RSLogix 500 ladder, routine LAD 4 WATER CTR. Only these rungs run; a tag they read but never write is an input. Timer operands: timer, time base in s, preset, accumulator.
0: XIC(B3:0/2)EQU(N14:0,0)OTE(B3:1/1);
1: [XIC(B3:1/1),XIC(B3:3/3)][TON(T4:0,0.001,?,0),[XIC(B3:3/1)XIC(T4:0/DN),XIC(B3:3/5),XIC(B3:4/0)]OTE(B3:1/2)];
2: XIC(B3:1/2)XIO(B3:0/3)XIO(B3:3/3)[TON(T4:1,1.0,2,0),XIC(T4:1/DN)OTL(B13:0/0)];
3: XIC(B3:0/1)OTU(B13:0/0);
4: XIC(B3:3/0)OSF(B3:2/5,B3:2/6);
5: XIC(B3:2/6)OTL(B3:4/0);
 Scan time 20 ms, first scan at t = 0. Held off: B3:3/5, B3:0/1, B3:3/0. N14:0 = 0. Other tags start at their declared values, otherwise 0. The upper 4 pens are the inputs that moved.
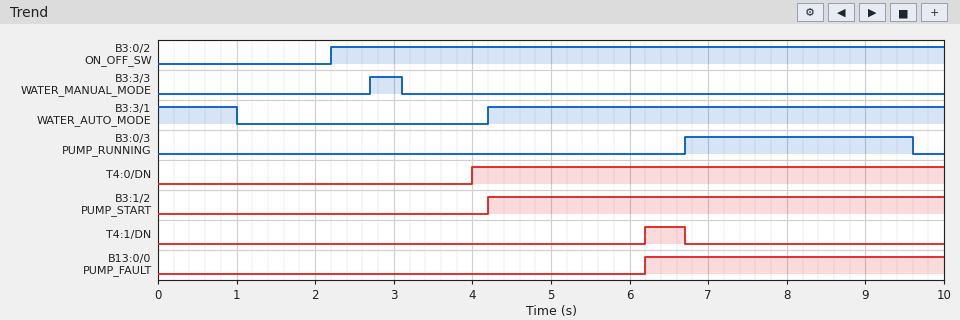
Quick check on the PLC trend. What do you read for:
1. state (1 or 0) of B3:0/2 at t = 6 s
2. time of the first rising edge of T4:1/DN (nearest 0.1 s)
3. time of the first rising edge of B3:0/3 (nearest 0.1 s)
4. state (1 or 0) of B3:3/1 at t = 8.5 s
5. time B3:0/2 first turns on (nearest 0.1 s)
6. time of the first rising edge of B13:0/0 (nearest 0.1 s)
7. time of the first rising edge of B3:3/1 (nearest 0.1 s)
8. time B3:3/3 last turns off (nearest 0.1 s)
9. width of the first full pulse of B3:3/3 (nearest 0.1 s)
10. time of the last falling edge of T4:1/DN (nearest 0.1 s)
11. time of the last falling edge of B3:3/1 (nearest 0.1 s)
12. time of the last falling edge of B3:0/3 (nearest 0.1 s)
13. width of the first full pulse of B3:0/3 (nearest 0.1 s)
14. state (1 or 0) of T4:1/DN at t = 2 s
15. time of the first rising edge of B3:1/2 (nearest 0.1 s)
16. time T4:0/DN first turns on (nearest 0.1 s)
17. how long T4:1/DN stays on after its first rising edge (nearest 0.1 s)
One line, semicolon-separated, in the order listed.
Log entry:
1; 6.2 s; 6.7 s; 1; 2.2 s; 6.2 s; 4.2 s; 3.1 s; 0.4 s; 6.7 s; 1.0 s; 9.6 s; 2.9 s; 0; 4.2 s; 4.0 s; 0.5 s
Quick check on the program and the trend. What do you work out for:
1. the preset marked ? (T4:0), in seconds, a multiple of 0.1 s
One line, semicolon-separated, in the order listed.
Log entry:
1.8 s
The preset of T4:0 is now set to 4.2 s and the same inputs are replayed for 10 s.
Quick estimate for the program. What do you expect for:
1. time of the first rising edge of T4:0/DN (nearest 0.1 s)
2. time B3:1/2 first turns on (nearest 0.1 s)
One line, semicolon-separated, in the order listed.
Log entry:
6.4 s; 6.4 s
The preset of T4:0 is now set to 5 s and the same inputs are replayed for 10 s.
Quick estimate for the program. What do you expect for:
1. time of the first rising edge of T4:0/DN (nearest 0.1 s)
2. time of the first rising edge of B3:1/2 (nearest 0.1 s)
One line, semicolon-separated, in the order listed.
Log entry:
7.2 s; 7.2 s
